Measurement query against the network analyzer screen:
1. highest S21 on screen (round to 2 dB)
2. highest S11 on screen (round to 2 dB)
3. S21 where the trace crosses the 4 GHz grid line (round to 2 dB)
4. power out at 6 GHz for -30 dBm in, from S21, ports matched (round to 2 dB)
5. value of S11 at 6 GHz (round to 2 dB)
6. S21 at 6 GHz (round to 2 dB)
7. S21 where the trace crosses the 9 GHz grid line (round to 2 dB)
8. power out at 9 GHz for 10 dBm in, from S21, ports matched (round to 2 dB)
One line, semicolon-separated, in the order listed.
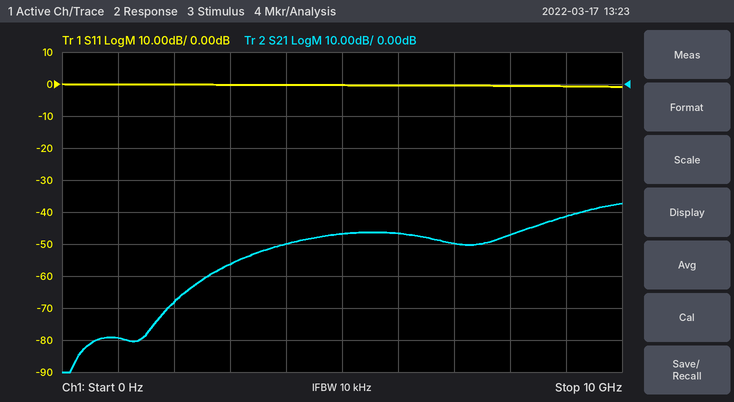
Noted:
-38 dB; 0 dB; -50 dB; -76 dBm; 0 dB; -46 dB; -42 dB; -32 dBm
